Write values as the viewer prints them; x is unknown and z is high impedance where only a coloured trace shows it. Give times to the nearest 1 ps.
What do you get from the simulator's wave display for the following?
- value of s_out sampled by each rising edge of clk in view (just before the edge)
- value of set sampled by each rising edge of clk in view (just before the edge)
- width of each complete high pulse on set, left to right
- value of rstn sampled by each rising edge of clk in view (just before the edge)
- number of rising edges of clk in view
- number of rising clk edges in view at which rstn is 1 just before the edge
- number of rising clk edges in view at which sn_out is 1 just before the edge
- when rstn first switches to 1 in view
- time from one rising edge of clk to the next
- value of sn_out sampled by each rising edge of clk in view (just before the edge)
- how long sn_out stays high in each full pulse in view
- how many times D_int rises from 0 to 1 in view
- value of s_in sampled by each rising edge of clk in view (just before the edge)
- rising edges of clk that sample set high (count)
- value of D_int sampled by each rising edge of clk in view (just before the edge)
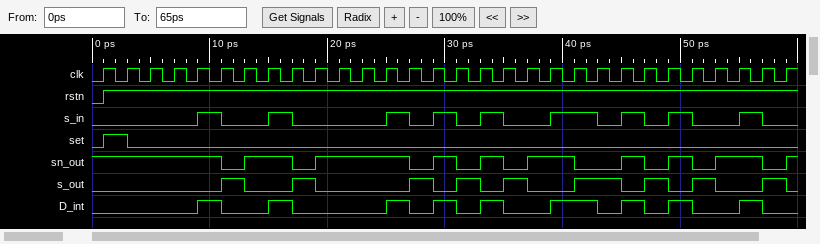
0 0 0 0 0 0 1 0 0 1 0 0 0 0 1 0 1 0 1 0 0 1 1 0 1 0 1 0 0 1
0 1 0 0 0 0 0 0 0 0 0 0 0 0 0 0 0 0 0 0 0 0 0 0 0 0 0 0 0 0
2 ps
0 1 1 1 1 1 1 1 1 1 1 1 1 1 1 1 1 1 1 1 1 1 1 1 1 1 1 1 1 1
30
29
20
1 ps
2 ps
1 1 1 1 1 1 0 1 1 0 1 1 1 1 0 1 0 1 0 1 1 0 0 1 0 1 0 1 1 0
4 ps, 8 ps, 2 ps, 2 ps, 4 ps, 2 ps, 2 ps, 4 ps
9
0 0 0 0 0 1 0 0 1 0 0 0 0 1 0 1 0 1 0 0 1 1 0 1 0 1 0 0 1 0
1
0 0 0 0 0 1 0 0 1 0 0 0 0 1 0 1 0 1 0 0 1 1 0 1 0 1 0 0 1 0
